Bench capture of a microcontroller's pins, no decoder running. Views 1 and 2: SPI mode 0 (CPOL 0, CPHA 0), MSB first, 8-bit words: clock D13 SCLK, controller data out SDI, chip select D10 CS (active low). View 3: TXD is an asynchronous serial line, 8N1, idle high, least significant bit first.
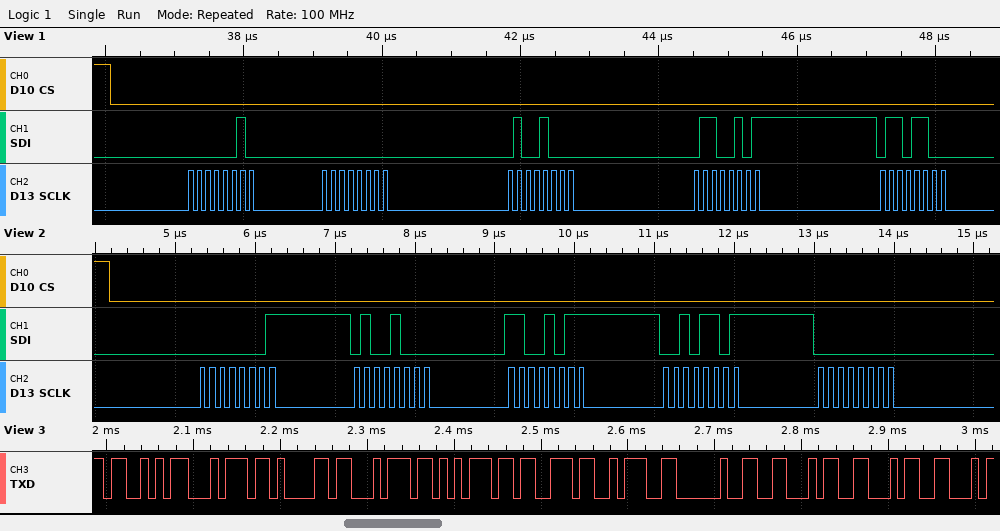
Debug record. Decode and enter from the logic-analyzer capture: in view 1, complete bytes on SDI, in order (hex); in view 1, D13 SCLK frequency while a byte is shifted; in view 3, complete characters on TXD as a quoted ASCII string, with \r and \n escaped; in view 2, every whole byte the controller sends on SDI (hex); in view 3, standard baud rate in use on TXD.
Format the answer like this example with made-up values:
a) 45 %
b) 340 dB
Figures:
a) 02 00 48 65 6C
b) 8 MHz
c) "Status: FFF"
d) 01 48 CB 2D 00
e) 115200 baud
